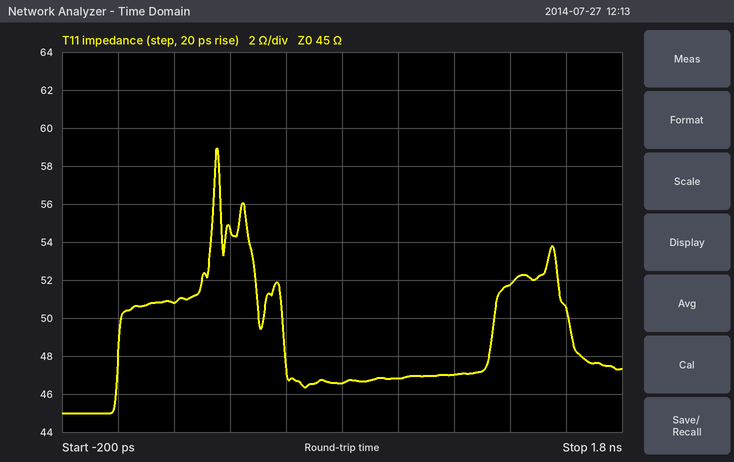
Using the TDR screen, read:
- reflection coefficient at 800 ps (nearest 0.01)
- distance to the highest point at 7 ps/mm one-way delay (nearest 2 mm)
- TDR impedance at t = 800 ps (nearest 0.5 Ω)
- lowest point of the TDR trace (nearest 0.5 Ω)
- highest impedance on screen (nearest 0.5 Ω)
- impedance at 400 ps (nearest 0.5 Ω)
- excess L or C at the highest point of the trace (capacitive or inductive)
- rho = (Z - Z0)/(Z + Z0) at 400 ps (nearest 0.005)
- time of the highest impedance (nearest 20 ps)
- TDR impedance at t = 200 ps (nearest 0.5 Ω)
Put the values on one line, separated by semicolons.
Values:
+0.02; 26 mm; 46.5 Ω; 45.0 Ω; 59.0 Ω; 54.5 Ω; inductive; +0.095; 360 ps; 51.0 Ω
